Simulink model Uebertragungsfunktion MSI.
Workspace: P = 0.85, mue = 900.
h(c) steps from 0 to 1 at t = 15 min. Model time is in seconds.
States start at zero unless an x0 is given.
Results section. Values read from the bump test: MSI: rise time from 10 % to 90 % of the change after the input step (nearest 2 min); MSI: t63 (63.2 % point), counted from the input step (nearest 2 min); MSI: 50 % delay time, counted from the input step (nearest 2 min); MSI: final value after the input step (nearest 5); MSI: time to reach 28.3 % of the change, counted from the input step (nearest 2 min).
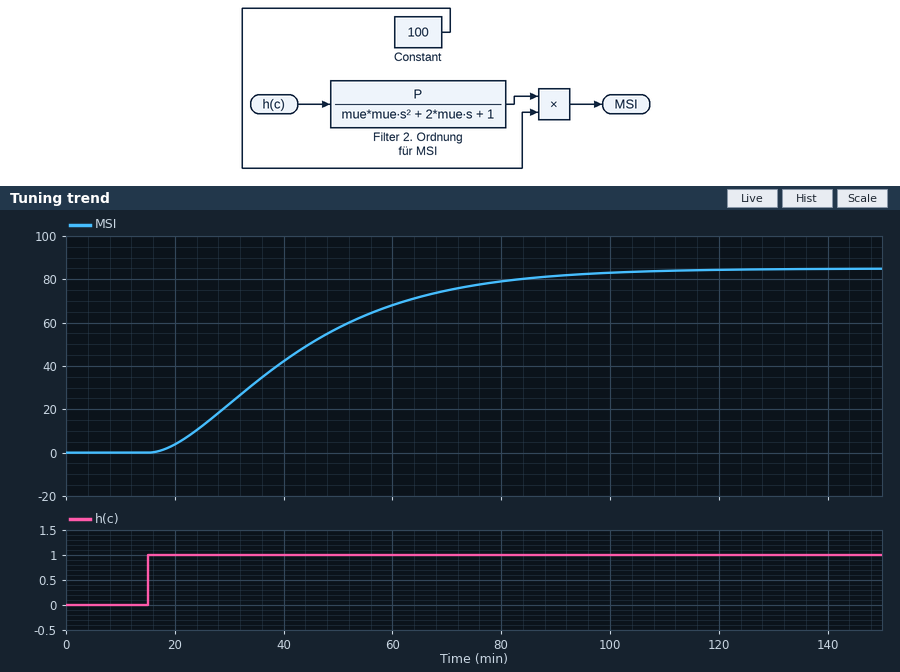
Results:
50 min
32 min
26 min
85
16 min
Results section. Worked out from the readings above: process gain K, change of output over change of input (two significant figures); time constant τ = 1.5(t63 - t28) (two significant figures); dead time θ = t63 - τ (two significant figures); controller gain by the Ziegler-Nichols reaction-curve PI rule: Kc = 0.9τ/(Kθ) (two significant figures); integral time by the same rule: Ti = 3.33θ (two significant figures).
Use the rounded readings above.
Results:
85
24 min
8.0 min
0.032
27 min
